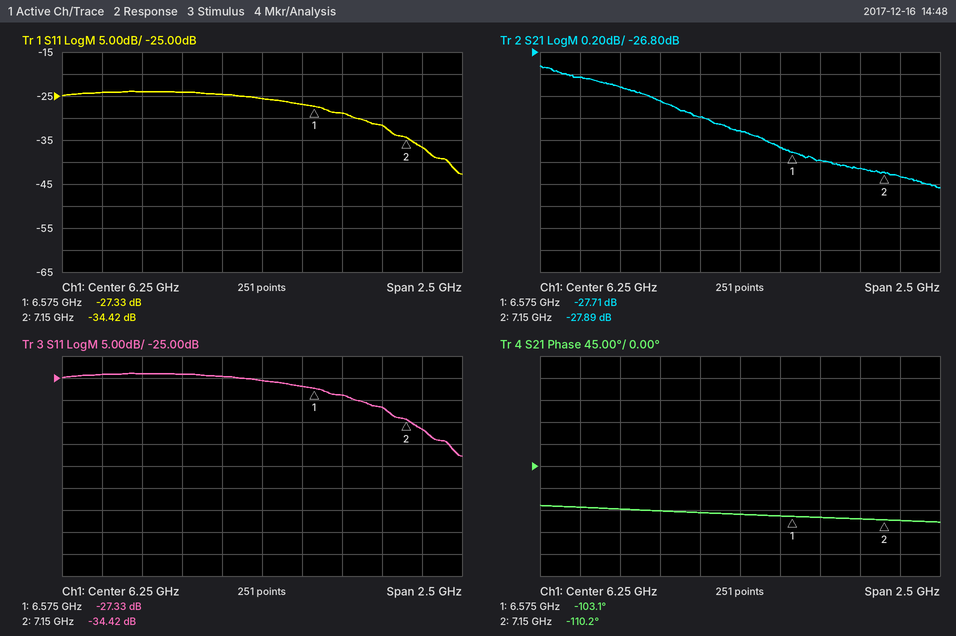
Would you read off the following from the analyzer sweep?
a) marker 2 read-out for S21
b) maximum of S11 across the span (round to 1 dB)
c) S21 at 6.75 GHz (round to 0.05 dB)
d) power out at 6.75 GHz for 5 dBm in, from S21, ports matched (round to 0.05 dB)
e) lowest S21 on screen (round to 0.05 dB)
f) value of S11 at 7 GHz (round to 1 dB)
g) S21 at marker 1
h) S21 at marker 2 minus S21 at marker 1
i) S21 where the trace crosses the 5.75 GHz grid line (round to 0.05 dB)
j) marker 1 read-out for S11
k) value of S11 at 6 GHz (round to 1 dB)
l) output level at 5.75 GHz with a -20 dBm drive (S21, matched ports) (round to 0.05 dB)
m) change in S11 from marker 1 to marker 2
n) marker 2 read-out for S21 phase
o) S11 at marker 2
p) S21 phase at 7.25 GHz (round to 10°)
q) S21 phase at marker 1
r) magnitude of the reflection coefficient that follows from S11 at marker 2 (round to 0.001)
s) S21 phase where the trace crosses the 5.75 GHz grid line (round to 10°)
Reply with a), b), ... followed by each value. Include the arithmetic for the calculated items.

a) -27.89 dB
b) -24 dB
c) -27.80 dB
d) 5 dBm + (-27.80 dB) = -22.80 dBm
e) -28.05 dB
f) -32 dB
g) -27.71 dB
h) -27.89 − (-27.71) = -0.18 dB
i) -27.25 dB
j) -27.33 dB
k) -25 dB
l) -20 dBm + (-27.25 dB) = -47.25 dBm
m) -34.42 − (-27.33) = -7.09 dB
n) -110.2°
o) -34.42 dB
p) -110°
q) -103.1°
r) 10^(-34.42/20) ≈ 0.019
s) -90°
